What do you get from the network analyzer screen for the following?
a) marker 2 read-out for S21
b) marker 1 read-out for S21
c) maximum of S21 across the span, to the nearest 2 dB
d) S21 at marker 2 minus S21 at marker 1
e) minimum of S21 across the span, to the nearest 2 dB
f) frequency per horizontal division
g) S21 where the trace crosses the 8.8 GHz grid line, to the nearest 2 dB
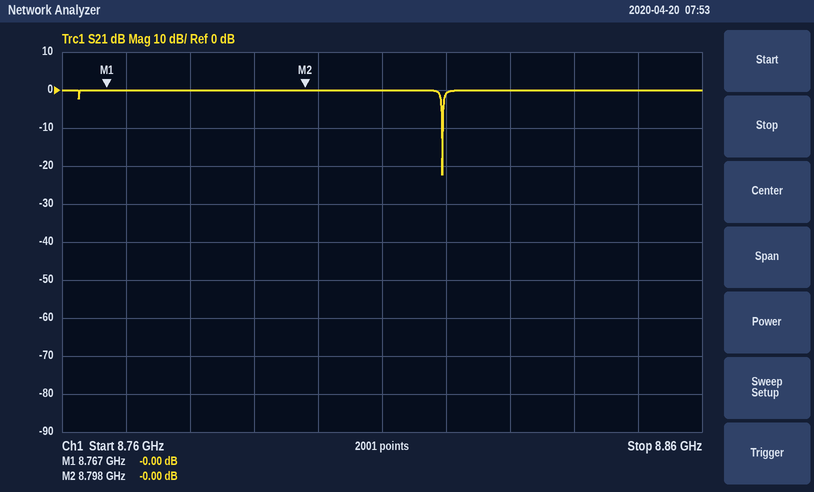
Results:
-0.00 dB
-0.00 dB
0 dB
0.00 dB
-22 dB
10 MHz
0 dB
